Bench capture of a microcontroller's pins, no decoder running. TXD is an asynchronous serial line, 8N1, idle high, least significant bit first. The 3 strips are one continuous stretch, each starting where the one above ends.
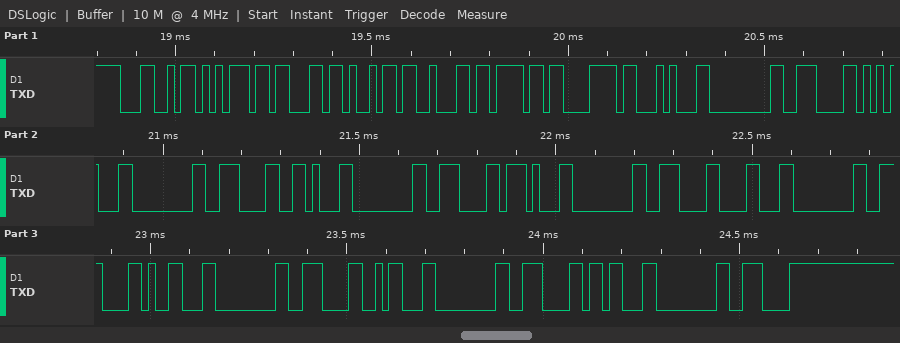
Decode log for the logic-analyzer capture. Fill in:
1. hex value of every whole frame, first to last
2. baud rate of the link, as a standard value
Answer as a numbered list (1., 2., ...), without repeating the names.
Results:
1. 0x4C 0x75 0x63 0x69 0x62 0x6F 0x78 0x14 0x00 0x0E 0x15 0x00 0x0E 0x16 0x00 0x0E 0x17 0x00 0x0E 0x18 0x00 0x0E 0x19 0x00 0x0E 0x1A 0x00 0x0E 0x1B 0x00 0x0E
2. 57600 baud
